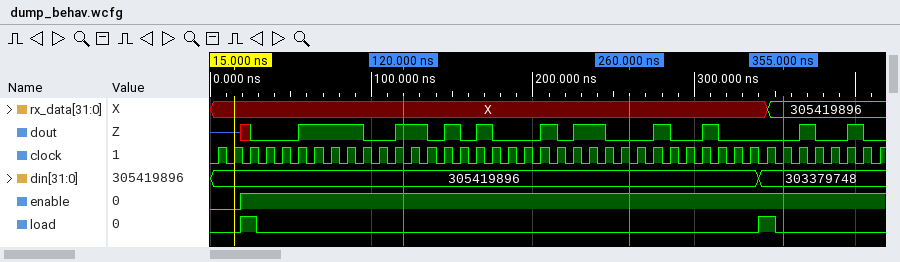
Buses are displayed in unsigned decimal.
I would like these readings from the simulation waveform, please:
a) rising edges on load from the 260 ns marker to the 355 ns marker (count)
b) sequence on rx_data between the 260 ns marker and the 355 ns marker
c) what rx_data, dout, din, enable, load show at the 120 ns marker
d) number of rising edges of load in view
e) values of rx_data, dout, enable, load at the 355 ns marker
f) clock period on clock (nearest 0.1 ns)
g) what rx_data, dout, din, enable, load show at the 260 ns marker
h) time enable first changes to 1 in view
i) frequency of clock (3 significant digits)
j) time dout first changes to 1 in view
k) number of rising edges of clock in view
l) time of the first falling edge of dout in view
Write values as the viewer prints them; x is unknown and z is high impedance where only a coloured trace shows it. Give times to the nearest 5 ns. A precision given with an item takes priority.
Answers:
1
X, 305419896
rx_data=X, dout=1, din=305419896, enable=1, load=0
2
rx_data=305419896, dout=0, enable=1, load=0
10 ns
rx_data=X, dout=0, din=305419896, enable=1, load=0
20 ns
100 MHz
55 ns
42
95 ns
